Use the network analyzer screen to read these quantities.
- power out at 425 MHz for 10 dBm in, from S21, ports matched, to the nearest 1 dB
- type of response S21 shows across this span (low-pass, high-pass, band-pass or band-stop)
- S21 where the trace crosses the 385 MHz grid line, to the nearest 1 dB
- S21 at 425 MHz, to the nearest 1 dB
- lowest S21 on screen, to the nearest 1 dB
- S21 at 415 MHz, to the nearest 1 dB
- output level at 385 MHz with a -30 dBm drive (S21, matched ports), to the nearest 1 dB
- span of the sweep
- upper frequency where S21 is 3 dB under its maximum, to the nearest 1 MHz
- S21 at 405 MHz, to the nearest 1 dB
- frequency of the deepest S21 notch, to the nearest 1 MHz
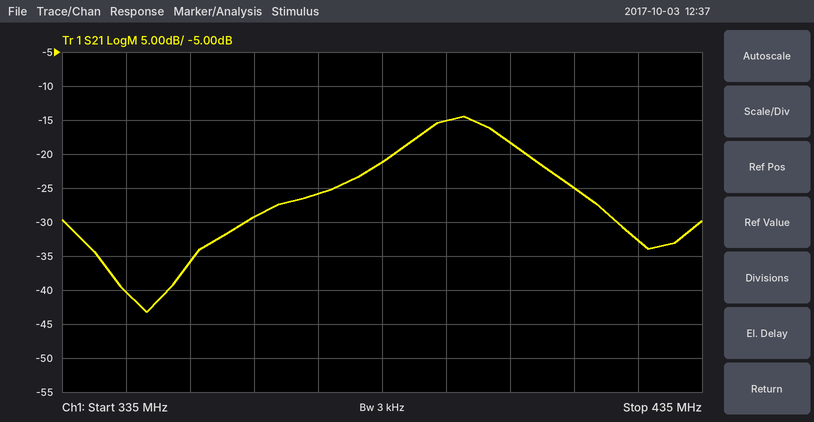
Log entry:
-23 dBm
band-pass
-21 dB
-33 dB
-43 dB
-25 dB
-51 dBm
100 MHz
404 MHz
-18 dB
348 MHz
